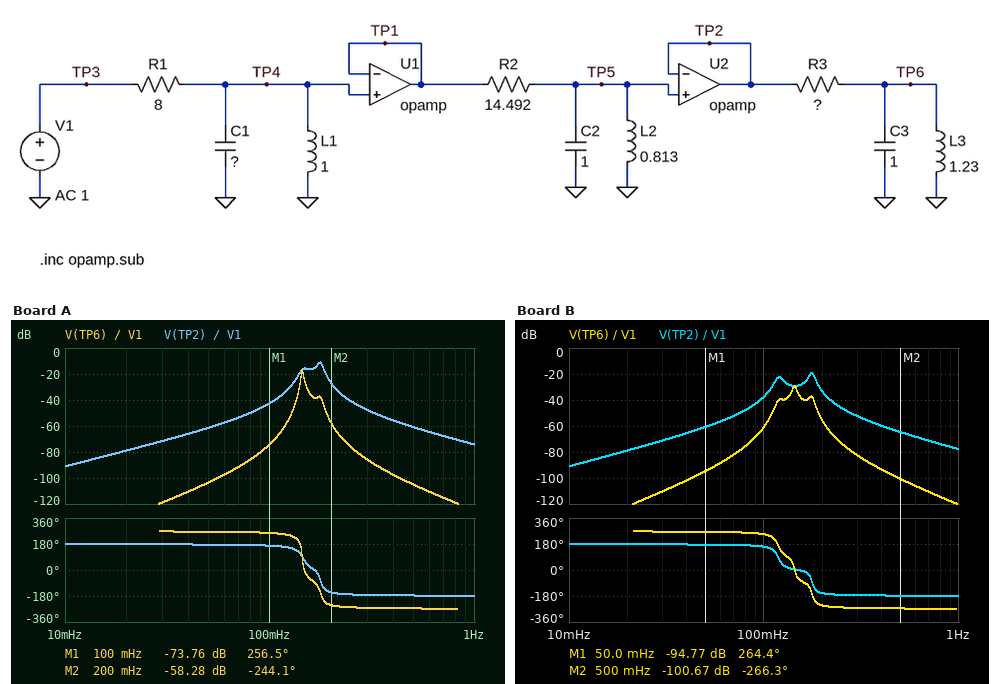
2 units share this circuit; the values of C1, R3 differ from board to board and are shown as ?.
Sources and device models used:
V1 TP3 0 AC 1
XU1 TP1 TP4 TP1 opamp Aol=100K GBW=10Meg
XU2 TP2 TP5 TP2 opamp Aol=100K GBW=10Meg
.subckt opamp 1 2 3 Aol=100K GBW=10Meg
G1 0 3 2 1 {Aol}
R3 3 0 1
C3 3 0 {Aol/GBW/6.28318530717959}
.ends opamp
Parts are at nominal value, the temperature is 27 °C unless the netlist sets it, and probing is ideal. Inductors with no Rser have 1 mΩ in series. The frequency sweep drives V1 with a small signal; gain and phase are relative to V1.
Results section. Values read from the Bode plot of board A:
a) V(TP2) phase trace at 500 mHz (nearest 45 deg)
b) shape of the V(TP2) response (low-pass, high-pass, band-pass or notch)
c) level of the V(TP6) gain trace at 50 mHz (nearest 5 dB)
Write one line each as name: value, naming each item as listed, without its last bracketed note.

V(TP2) phase trace at 500 mHz: -180 deg
shape of the V(TP2) response: band-pass
level of the V(TP6) gain trace at 50 mHz: -105 dB
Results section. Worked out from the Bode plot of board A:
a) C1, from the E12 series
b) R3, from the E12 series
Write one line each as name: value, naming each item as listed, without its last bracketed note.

C1, from the E12 series: 1.2 F
R3, from the E12 series: 56 Ω
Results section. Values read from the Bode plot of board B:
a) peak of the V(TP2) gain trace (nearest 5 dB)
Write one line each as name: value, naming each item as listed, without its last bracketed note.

peak of the V(TP2) gain trace: -20 dB
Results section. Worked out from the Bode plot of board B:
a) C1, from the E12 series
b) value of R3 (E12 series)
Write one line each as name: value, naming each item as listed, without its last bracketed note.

C1, from the E12 series: 1.8 F
value of R3: 22 Ω
